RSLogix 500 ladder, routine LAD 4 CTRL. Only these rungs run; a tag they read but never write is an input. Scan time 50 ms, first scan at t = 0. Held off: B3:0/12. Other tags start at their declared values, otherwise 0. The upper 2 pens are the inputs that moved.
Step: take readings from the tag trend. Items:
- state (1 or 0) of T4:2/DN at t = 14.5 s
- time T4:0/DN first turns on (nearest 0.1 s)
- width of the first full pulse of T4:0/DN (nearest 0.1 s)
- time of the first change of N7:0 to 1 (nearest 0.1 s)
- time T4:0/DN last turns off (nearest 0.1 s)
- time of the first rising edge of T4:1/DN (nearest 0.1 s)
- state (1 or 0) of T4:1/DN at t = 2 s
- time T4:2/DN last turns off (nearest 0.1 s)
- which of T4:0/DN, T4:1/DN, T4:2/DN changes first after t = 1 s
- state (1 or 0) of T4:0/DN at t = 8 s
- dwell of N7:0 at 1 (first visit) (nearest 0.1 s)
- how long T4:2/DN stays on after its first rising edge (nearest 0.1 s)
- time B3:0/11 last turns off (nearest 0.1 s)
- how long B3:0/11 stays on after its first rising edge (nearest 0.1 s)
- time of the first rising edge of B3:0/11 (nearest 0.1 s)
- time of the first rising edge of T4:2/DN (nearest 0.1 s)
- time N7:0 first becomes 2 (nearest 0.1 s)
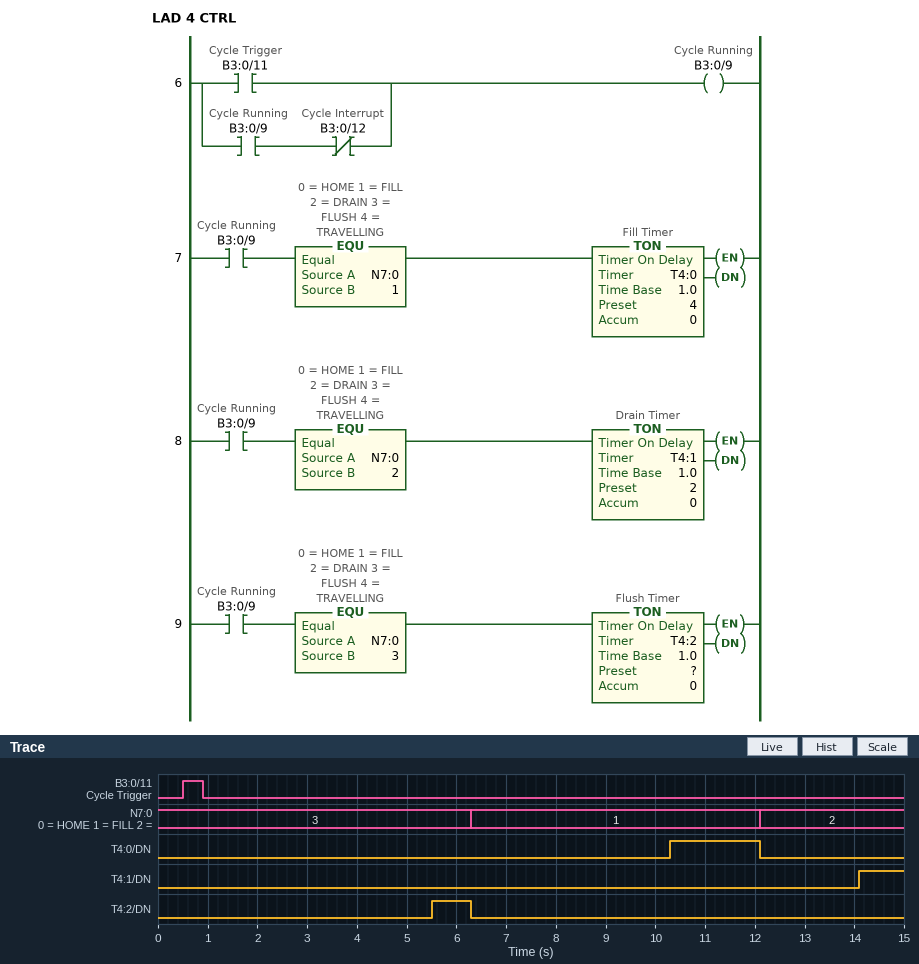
0
10.3 s
1.8 s
6.3 s
12.1 s
14.1 s
0
6.3 s
T4:2/DN
0
5.8 s
0.8 s
0.9 s
0.4 s
0.5 s
5.5 s
12.1 s
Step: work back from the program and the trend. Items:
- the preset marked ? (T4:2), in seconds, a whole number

5 s
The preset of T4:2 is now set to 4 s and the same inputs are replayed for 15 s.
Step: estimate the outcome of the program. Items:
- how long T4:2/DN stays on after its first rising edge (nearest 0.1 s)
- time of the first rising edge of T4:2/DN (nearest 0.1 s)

1.8 s
4.5 s
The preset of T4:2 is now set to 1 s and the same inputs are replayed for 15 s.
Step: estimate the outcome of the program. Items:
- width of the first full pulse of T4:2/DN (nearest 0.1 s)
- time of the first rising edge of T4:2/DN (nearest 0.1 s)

4.8 s
1.5 s
